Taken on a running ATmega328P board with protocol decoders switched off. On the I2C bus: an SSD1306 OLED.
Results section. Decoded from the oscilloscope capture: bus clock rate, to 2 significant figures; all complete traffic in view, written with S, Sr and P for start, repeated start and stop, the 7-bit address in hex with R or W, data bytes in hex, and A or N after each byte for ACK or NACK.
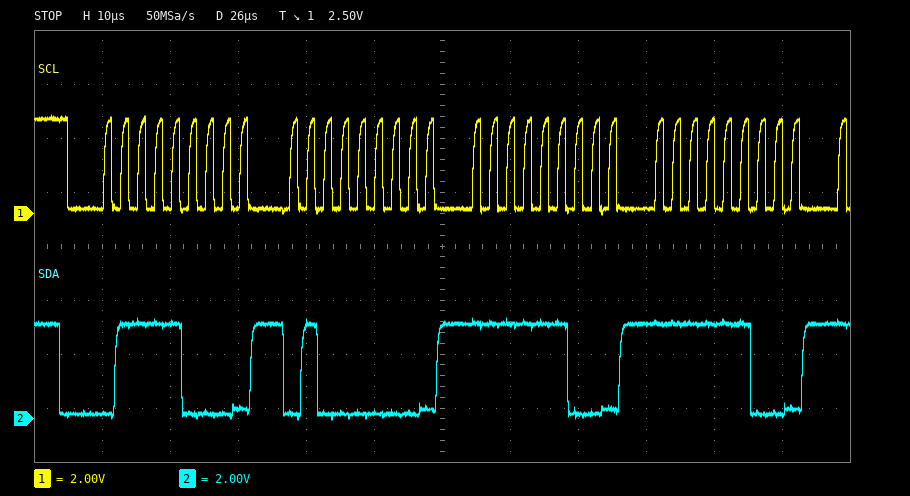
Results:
400 kHz
S 3CW A 40 A FC A FC A
